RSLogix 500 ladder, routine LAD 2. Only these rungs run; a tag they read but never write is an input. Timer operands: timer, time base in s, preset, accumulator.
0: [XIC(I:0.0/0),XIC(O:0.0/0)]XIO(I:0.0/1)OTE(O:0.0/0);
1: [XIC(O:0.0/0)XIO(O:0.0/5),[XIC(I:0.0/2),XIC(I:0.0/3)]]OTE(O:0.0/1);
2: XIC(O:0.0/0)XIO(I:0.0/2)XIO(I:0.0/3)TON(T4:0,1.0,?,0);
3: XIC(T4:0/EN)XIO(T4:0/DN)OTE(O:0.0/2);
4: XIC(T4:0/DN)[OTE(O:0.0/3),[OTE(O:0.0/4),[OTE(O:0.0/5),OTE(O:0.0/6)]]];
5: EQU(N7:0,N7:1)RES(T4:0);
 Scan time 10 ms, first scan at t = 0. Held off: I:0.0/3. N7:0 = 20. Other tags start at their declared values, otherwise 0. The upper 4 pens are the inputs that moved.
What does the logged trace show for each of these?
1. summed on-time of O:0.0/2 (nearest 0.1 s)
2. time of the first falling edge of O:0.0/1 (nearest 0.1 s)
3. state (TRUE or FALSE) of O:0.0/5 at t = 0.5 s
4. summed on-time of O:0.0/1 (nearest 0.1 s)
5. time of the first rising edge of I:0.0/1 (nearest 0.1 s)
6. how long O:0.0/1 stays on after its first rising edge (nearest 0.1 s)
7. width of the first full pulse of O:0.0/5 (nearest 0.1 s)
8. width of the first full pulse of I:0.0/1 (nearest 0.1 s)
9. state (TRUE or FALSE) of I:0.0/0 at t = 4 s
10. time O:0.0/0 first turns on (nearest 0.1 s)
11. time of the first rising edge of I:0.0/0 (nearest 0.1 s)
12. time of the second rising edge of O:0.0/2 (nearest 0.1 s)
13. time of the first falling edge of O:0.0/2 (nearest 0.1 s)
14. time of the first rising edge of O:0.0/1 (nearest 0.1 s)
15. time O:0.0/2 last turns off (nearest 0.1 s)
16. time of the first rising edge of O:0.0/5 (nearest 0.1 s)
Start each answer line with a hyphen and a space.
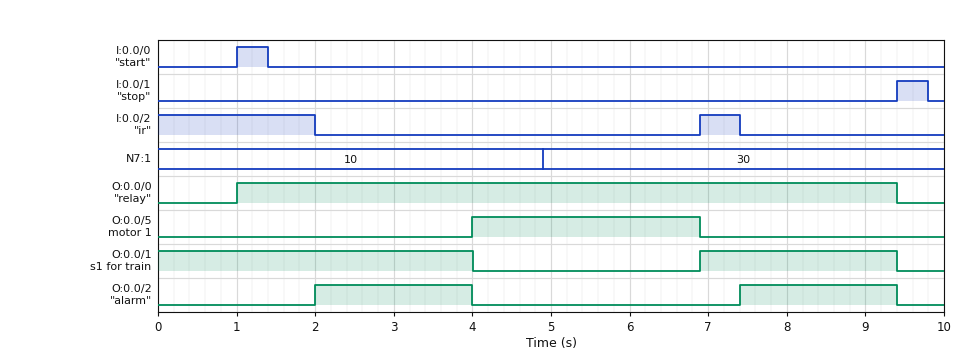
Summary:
- 4.0 s
- 4.0 s
- FALSE
- 6.5 s
- 9.4 s
- 2.5 s
- 2.9 s
- 0.4 s
- FALSE
- 1.0 s
- 1.0 s
- 7.4 s
- 4.0 s
- 6.9 s
- 9.4 s
- 4.0 s
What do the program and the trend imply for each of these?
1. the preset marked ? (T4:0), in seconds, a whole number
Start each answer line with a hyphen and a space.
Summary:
- 2 s
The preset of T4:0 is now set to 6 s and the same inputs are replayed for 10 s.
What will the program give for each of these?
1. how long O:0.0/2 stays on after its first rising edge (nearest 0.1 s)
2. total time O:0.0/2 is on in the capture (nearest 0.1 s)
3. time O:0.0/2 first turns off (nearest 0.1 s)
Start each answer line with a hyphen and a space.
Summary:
- 4.9 s
- 6.9 s
- 6.9 s
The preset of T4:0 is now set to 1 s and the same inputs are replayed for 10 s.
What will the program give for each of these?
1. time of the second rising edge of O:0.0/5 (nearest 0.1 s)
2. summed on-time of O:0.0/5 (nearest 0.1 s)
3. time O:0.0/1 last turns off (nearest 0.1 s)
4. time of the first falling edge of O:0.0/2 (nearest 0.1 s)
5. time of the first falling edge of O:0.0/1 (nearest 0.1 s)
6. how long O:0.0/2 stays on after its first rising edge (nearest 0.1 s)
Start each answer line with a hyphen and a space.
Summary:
- 8.4 s
- 4.9 s
- 8.4 s
- 3.0 s
- 3.0 s
- 1.0 s
